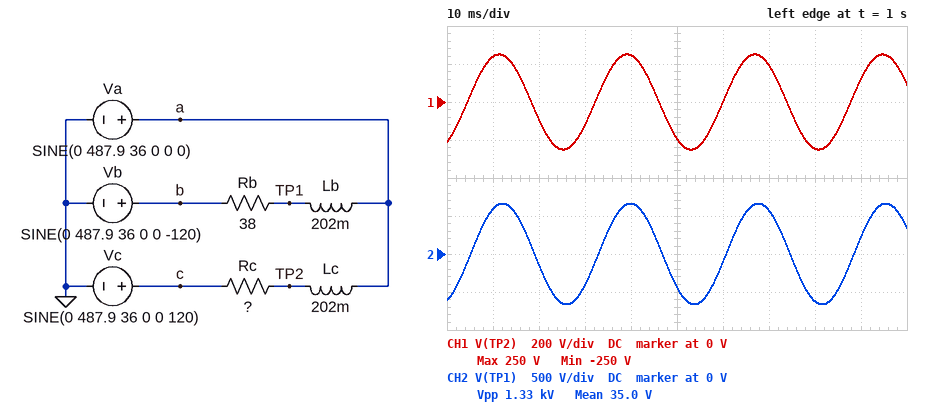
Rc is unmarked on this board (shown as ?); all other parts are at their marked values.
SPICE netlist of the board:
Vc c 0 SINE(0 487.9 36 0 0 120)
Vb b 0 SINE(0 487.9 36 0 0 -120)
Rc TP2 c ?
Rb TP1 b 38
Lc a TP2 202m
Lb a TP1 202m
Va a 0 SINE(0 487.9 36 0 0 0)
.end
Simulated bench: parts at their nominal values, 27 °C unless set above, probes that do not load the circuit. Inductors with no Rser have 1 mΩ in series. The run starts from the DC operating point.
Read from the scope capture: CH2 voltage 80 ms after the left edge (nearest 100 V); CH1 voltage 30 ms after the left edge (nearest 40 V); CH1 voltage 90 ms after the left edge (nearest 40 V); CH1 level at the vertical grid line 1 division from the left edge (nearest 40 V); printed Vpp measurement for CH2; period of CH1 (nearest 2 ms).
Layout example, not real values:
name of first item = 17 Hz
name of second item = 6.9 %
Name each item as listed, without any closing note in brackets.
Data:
CH2 voltage 80 ms after the left edge = -600 V
CH1 voltage 30 ms after the left edge = -120 V
CH1 voltage 90 ms after the left edge = 120 V
CH1 level at the vertical grid line 1 division from the left edge = 240 V
printed Vpp measurement for CH2 = 1.33 kV
period of CH1 = 28 ms
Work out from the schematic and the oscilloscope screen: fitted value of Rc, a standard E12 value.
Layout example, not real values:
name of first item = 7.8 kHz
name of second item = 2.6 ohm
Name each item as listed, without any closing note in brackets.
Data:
fitted value of Rc, a standard E12 value = 82 Ω
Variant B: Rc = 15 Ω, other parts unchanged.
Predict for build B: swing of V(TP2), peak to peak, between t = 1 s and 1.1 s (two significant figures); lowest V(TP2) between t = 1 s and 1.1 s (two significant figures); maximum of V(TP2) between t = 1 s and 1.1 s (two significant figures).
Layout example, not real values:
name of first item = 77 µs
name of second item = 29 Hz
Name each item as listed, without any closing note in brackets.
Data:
swing of V(TP2), peak to peak, between t = 1 s and 1.1 s = 680 V
lowest V(TP2) between t = 1 s and 1.1 s = -340 V
maximum of V(TP2) between t = 1 s and 1.1 s = 340 V
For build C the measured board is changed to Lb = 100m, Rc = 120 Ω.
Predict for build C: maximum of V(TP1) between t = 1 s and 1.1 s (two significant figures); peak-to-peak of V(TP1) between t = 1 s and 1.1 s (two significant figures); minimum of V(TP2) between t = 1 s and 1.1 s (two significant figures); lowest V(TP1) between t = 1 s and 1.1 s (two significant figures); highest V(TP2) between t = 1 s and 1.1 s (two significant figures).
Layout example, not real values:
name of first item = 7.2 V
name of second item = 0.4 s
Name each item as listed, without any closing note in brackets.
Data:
maximum of V(TP1) between t = 1 s and 1.1 s = 650 V
peak-to-peak of V(TP1) between t = 1 s and 1.1 s = 1.3 kV
minimum of V(TP2) between t = 1 s and 1.1 s = -320 V
lowest V(TP1) between t = 1 s and 1.1 s = -650 V
highest V(TP2) between t = 1 s and 1.1 s = 320 V
